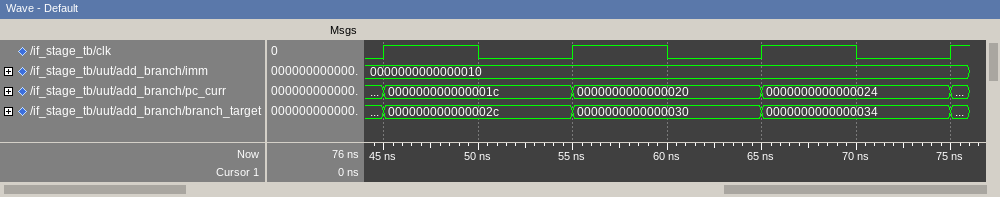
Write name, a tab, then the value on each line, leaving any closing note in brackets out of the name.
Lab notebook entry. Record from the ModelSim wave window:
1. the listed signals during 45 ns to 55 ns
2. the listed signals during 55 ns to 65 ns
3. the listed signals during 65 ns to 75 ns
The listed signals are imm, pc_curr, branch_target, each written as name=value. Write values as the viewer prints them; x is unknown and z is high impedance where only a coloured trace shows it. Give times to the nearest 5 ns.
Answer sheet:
the listed signals during 45 ns to 55 ns	imm=0000000000000010, pc_curr=000000000000001c, branch_target=000000000000002c
the listed signals during 55 ns to 65 ns	imm=0000000000000010, pc_curr=0000000000000020, branch_target=0000000000000030
the listed signals during 65 ns to 75 ns	imm=0000000000000010, pc_curr=0000000000000024, branch_target=0000000000000034
